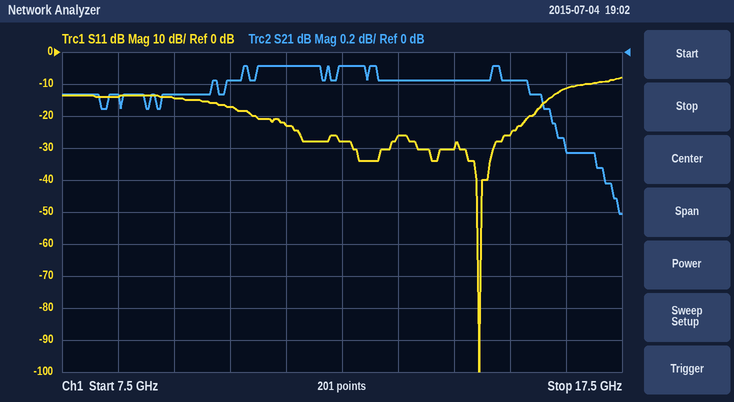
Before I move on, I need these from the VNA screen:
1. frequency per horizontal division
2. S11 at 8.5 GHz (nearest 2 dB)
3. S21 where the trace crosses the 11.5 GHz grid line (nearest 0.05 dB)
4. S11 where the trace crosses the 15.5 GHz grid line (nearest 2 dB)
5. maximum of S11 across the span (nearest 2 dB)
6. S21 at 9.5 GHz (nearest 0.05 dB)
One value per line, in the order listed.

1 GHz
-14 dB
-0.10 dB
-26 dB
-8 dB
-0.25 dB
